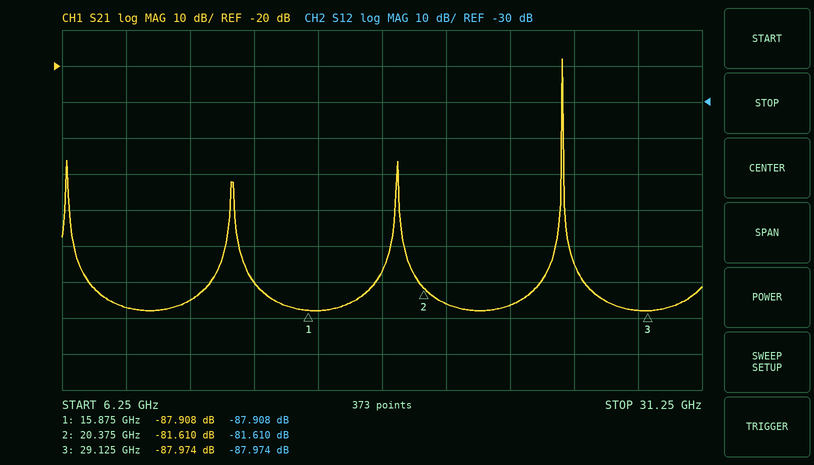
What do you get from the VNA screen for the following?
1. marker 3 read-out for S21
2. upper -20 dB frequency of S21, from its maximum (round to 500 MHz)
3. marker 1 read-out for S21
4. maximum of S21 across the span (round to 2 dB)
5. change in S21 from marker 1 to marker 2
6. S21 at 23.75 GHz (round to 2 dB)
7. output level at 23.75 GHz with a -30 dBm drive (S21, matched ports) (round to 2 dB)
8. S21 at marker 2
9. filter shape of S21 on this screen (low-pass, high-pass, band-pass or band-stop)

-87.974 dB
26.0 GHz
-87.908 dB
-18 dB
6.298 dB
-86 dB
-116 dBm
-81.610 dB
band-pass
